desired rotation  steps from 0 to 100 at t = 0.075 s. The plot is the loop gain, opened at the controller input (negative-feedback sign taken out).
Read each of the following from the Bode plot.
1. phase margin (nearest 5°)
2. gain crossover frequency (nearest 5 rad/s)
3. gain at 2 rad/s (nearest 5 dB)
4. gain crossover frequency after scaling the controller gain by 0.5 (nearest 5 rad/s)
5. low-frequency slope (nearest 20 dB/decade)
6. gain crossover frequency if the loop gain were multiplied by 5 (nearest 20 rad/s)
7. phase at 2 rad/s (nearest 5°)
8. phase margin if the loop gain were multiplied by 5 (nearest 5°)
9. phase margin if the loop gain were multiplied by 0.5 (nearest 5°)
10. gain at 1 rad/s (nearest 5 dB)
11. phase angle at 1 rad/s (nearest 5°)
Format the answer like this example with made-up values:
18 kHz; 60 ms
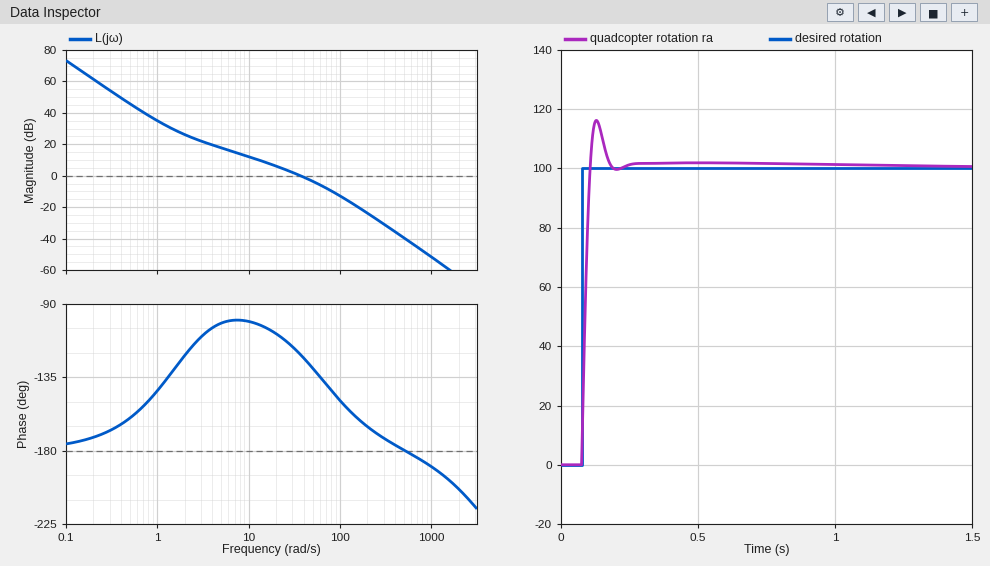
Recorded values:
60°; 35 rad/s; 25 dB; 20 rad/s; -40 dB/decade; 100 rad/s; -120°; 30°; 70°; 35 dB; -145°
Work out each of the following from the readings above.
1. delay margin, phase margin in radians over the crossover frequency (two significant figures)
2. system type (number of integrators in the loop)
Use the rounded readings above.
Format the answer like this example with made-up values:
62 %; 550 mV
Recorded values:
0.030 s; 2
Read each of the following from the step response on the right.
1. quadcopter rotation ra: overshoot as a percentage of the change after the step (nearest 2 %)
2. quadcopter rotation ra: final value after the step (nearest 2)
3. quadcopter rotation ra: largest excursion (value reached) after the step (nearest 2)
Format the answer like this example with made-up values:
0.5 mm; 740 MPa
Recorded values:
16 %; 100; 116
